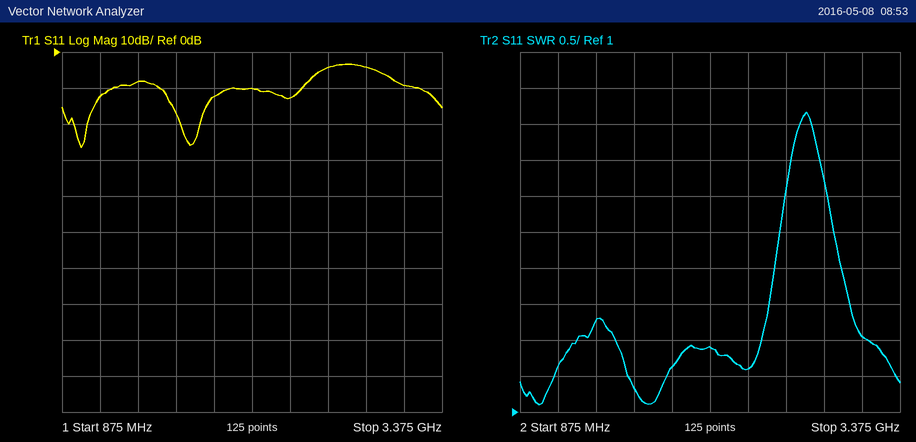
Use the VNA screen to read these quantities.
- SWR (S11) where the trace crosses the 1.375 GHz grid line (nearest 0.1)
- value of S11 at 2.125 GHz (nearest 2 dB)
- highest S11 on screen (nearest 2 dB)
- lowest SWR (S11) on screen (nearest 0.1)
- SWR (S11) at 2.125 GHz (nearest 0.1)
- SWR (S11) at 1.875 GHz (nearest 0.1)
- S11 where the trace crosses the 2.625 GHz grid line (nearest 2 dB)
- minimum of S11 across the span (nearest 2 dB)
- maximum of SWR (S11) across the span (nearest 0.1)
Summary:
2.3
-10 dB
-4 dB
1.1
1.9
1.6
-4 dB
-26 dB
5.2
